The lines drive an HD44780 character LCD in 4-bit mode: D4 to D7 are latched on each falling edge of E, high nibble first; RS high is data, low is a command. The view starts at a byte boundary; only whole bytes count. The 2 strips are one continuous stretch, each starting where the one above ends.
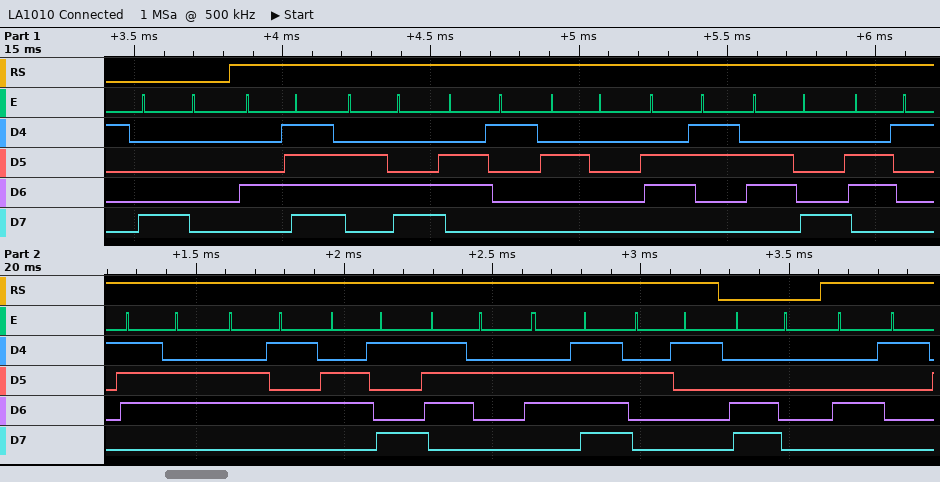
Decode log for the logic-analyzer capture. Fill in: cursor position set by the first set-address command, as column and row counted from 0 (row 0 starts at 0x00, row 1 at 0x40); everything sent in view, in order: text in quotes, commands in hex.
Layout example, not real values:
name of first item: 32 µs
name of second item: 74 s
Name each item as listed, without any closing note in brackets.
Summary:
cursor position set by the first set-address command, as column and row counted from 0: column 0, row 0
everything sent in view, in order: text in quotes, commands in hex: 0x80 "Ola chaveiro!" 0xC0 "A"
